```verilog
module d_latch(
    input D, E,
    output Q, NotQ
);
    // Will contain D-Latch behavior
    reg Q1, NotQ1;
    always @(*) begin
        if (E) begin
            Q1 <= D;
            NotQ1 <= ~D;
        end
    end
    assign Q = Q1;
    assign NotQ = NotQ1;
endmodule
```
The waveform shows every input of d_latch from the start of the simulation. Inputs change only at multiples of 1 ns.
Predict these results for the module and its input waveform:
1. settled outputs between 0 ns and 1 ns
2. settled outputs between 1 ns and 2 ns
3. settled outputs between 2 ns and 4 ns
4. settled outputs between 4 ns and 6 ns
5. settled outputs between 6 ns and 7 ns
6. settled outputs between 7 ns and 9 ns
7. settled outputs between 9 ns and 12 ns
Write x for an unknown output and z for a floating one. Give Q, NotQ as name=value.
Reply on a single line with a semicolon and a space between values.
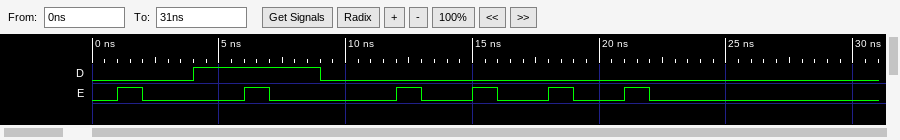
Q=x, NotQ=x; Q=0, NotQ=1; Q=0, NotQ=1; Q=0, NotQ=1; Q=1, NotQ=0; Q=1, NotQ=0; Q=1, NotQ=0
